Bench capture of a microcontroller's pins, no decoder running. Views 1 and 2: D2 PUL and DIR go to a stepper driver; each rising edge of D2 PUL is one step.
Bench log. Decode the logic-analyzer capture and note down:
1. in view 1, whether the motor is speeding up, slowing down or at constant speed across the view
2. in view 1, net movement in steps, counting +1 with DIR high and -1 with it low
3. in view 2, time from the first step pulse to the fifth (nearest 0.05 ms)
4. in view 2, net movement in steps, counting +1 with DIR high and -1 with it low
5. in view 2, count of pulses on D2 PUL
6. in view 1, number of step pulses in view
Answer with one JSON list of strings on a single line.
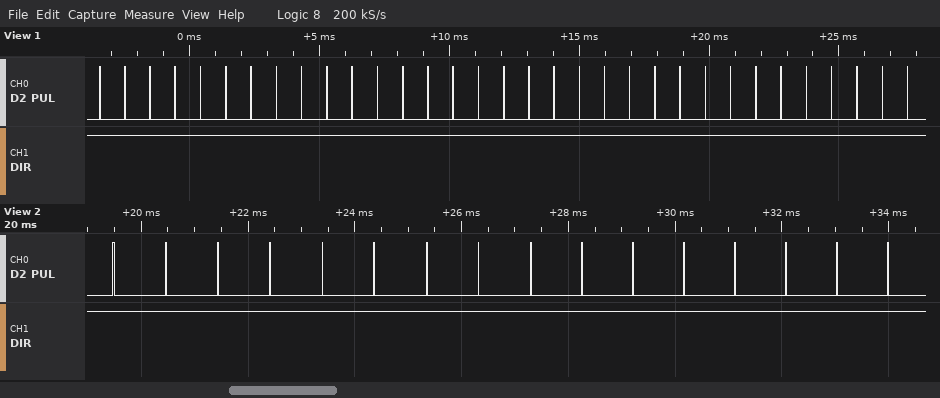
["constant speed", "+33", "3.90 ms", "+16", "16", "33"]
